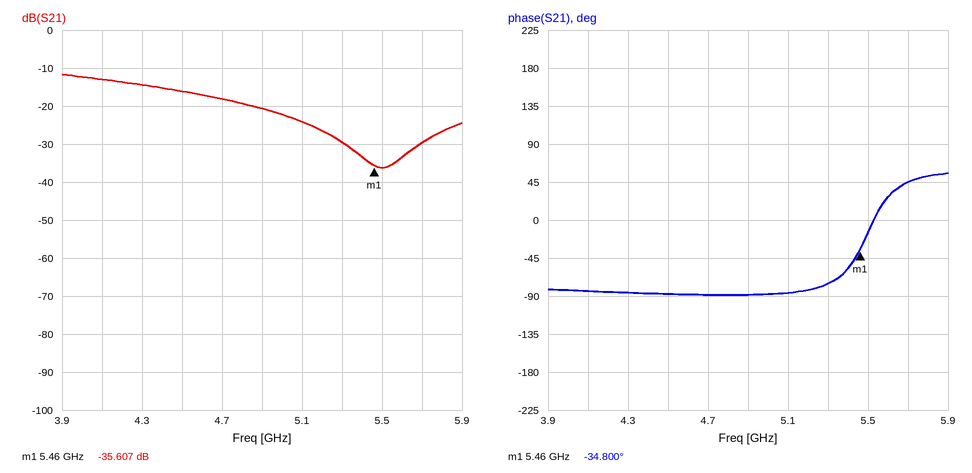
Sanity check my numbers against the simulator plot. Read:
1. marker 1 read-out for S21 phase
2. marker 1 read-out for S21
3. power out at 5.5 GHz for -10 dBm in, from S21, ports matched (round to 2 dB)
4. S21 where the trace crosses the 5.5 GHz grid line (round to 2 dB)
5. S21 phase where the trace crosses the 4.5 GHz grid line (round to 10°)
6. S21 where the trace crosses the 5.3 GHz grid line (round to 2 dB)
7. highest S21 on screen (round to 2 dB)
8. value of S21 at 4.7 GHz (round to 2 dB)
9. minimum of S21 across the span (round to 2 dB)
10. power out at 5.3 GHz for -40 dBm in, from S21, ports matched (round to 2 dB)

-34.800°
-35.607 dB
-46 dBm
-36 dB
-90°
-30 dB
-12 dB
-18 dB
-36 dB
-70 dBm
